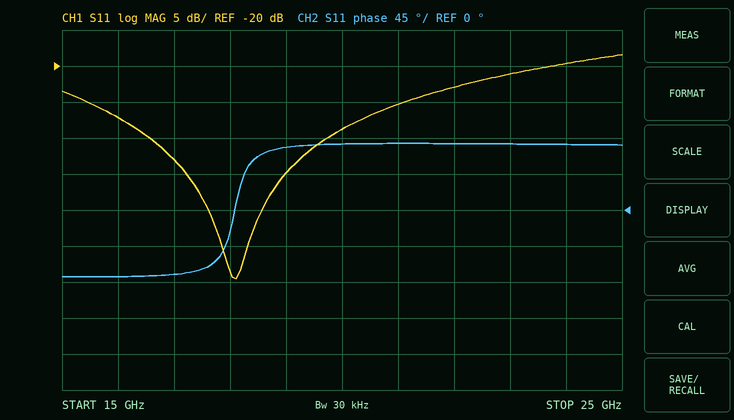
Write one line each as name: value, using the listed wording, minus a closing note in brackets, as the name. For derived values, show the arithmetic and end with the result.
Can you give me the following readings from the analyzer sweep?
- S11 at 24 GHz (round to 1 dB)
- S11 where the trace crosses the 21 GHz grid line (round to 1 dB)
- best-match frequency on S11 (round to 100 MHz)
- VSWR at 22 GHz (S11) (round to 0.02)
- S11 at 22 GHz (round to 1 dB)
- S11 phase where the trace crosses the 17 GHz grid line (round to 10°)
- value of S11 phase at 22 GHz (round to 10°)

S11 at 24 GHz: -20 dB
S11 where the trace crosses the 21 GHz grid line: -25 dB
best-match frequency on S11: 18.1 GHz
VSWR at 22 GHz (S11): |Γ| = 10^(-23/20) = 0.0708; VSWR = (1 + 0.0708)/(1 − 0.0708) ≈ 1.15, so 1.16 to the nearest 0.02
S11 at 22 GHz: -23 dB
S11 phase where the trace crosses the 17 GHz grid line: -80°
value of S11 phase at 22 GHz: 80°
